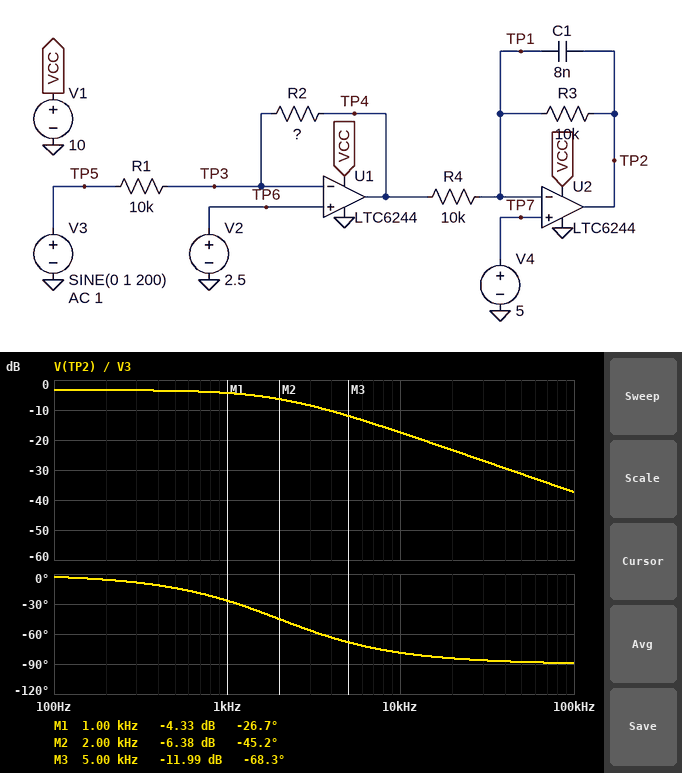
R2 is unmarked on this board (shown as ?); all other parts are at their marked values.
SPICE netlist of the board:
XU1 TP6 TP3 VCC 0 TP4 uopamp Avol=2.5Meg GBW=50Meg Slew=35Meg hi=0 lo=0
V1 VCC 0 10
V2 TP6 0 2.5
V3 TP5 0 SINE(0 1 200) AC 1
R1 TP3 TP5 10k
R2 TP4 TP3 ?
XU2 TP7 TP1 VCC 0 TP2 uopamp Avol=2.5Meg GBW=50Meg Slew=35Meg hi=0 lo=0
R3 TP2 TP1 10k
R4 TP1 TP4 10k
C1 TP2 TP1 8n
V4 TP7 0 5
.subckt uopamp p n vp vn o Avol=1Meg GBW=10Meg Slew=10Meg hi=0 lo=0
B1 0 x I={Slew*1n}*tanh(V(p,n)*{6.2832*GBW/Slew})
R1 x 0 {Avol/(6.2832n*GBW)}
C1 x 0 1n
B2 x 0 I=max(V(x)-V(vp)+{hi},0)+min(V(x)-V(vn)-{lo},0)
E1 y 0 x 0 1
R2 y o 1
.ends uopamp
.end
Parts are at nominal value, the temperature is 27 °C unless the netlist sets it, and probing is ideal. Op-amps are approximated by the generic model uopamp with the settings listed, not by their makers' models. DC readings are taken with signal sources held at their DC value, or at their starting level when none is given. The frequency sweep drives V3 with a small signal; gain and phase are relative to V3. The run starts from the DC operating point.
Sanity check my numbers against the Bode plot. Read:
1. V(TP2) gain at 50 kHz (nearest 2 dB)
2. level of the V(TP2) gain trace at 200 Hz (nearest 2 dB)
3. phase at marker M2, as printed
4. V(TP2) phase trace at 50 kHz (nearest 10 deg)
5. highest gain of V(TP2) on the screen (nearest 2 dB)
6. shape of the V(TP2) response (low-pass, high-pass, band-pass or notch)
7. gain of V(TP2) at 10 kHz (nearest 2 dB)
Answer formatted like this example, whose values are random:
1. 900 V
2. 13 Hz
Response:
1. -32 dB
2. -4 dB
3. -45.2 deg
4. -90 deg
5. -4 dB
6. low-pass
7. -18 dB
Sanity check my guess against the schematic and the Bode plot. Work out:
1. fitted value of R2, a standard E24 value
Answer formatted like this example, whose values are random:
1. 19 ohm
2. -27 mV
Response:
1. 6.8 kΩ
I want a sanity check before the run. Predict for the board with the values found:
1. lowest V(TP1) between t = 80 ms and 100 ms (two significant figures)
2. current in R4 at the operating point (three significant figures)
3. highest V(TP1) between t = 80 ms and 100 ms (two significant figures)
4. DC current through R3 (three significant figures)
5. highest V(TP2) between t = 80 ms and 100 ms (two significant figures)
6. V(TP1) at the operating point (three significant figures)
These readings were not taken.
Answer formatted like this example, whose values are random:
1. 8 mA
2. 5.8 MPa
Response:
1. 5.0 V
2. 80.0 µA
3. 5.0 V
4. 80.0 µA
5. 6.5 V
6. 5.00 V
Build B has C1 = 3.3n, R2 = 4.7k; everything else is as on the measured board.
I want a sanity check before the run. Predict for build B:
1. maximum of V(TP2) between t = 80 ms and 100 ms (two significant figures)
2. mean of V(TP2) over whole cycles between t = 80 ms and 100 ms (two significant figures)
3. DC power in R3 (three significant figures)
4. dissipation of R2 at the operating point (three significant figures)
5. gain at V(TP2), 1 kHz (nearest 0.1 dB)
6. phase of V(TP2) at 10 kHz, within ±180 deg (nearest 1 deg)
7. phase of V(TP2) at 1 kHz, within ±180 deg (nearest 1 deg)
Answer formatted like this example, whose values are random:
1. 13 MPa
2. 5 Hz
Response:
1. 6.8 V
2. 6.3 V
3. 176 µW
4. 294 µW
5. -6.7 dB
6. -64 deg
7. -12 deg
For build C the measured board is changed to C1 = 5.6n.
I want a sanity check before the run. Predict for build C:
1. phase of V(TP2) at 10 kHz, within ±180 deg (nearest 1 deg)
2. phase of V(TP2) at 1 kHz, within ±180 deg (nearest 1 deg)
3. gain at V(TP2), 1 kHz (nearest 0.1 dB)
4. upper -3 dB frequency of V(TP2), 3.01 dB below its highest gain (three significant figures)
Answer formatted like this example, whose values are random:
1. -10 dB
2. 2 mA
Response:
1. -74 deg
2. -19 deg
3. -3.9 dB
4. 2.84 kHz
